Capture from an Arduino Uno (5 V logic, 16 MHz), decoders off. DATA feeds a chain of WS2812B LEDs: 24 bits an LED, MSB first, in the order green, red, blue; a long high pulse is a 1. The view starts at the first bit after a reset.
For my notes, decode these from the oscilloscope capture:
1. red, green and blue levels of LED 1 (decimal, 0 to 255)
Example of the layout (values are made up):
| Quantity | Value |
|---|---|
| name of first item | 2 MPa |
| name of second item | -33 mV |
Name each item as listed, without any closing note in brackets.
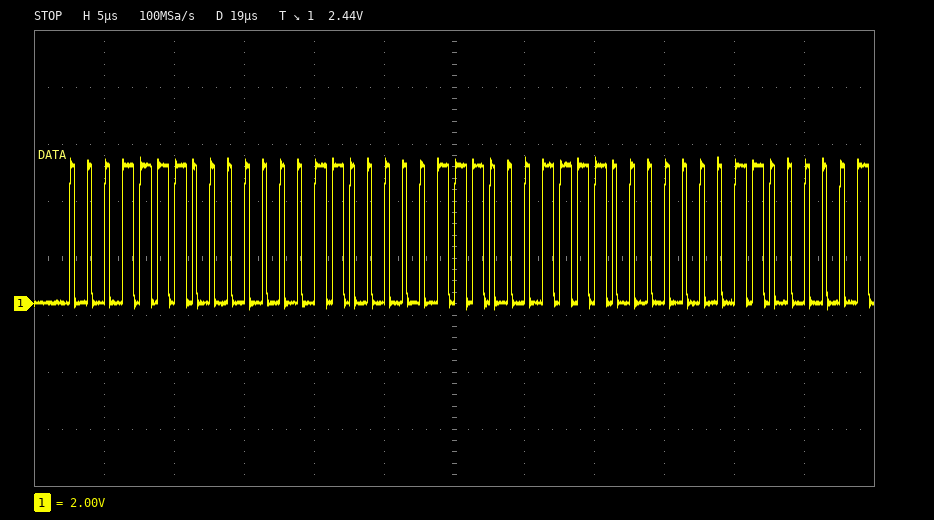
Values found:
| Quantity | Value |
|---|---|
| red, green and blue levels of LED 1 | 3, 30, 7 |
